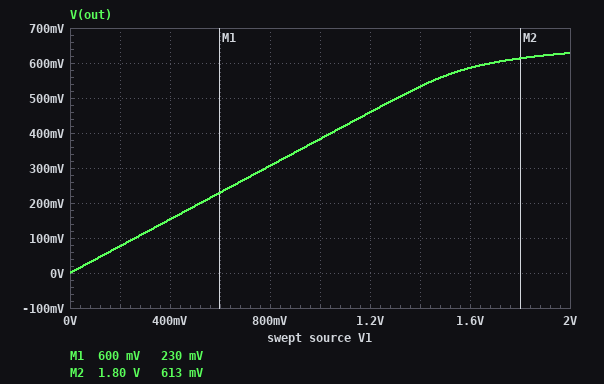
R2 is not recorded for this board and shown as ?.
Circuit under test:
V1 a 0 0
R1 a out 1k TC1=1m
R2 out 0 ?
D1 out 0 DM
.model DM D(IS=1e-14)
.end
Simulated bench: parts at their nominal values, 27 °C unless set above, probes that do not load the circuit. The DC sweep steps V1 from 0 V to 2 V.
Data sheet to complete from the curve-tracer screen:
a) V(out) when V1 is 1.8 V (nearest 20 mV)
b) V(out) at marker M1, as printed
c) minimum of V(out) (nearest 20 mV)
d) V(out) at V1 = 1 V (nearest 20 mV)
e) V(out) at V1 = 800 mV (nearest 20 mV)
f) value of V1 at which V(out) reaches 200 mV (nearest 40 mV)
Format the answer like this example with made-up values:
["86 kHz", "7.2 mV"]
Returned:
["620 mV", "230 mV", "0 V", "380 mV", "300 mV", "520 mV"]
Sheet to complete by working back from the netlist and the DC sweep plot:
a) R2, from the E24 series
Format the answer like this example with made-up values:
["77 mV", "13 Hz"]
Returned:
["620 Ω"]
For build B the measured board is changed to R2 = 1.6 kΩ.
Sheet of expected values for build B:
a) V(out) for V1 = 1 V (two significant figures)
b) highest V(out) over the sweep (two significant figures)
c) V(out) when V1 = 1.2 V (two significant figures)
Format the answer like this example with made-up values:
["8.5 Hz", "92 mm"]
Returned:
["580 mV", "650 mV", "610 mV"]
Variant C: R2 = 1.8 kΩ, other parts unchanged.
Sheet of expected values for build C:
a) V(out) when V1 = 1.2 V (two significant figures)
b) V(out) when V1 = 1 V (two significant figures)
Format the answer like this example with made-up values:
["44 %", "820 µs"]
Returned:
["620 mV", "590 mV"]
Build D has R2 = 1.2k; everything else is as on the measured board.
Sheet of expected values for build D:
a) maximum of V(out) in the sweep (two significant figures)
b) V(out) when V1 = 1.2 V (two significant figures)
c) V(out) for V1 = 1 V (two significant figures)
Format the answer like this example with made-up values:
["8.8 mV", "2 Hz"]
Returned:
["650 mV", "600 mV", "540 mV"]
